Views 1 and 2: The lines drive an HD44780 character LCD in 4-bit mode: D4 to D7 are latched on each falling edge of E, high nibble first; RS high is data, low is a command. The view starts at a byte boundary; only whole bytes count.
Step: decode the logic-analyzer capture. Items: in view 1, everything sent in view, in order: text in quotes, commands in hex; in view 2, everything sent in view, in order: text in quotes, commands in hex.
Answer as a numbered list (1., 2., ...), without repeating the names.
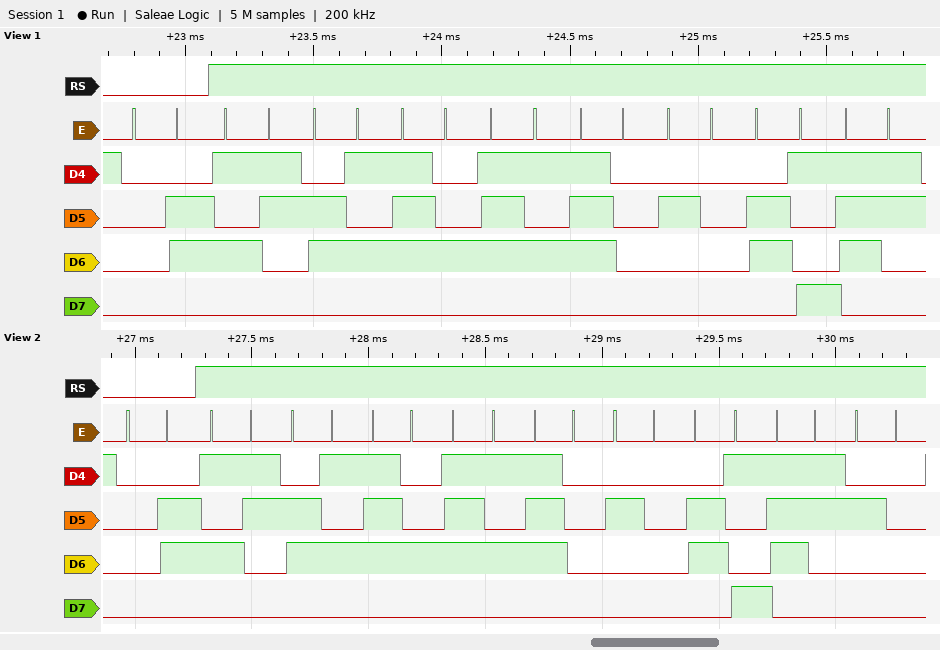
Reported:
1. 0x06 "Setup is"
2. 0x06 "Setup is "
